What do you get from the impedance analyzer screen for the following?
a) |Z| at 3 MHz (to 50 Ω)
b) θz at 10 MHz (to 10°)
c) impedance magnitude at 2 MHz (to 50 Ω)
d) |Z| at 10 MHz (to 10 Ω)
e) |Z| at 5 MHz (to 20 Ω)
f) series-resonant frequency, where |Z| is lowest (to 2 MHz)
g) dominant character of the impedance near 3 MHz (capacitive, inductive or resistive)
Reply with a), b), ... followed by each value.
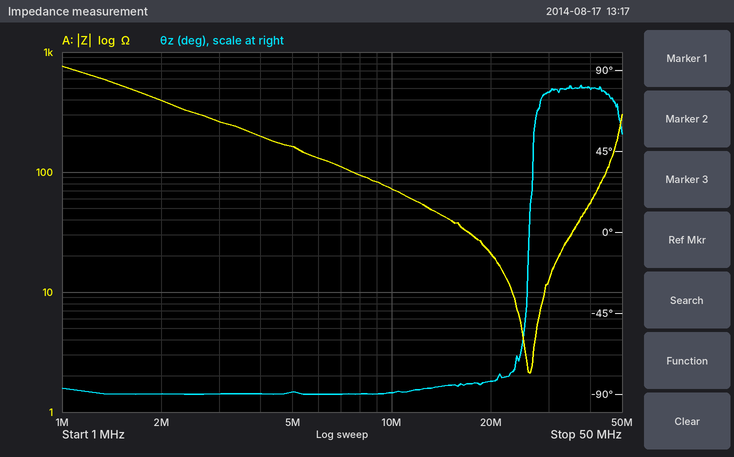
a) 250 Ω
b) -90°
c) 400 Ω
d) 70 Ω
e) 160 Ω
f) 26 MHz
g) capacitive
